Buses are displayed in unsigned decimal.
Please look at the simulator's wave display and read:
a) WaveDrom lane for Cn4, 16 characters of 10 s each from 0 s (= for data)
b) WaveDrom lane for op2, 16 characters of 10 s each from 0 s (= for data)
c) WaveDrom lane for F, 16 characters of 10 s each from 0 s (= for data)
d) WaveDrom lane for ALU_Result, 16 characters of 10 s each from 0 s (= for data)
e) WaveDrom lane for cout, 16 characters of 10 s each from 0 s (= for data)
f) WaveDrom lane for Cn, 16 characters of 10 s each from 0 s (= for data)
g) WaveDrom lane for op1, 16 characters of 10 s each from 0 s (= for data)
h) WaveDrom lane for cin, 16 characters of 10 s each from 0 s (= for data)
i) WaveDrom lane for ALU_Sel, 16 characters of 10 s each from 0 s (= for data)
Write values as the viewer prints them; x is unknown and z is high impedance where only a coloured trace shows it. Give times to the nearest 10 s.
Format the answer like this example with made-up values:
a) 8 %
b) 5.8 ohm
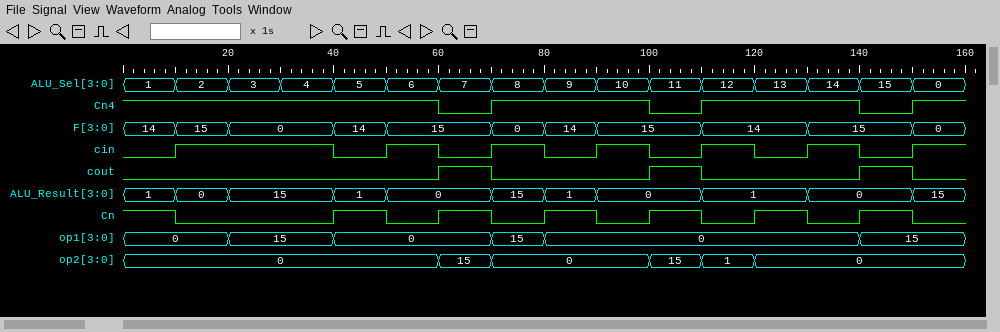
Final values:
a) {name: 'Cn4', wave: '1.....01..01..01'}
b) {name: 'op2', wave: '=.....==..===...', data: '0 15 0 15 1 0'}
c) {name: 'F', wave: '===.==.===.=.=.=', data: '14 15 0 14 15 0 14 15 14 15 0'}
d) {name: 'ALU_Result', wave: '===.==.===.=.=.=', data: '1 0 15 1 0 15 1 0 1 0 15'}
e) {name: 'cout', wave: '0.....10..10..10'}
f) {name: 'Cn', wave: '10..101010101010'}
g) {name: 'op1', wave: '=.=.=..==.....=.', data: '0 15 0 15 0 15'}
h) {name: 'cin', wave: '01..010101010101'}
i) {name: 'ALU_Sel', wave: '================', data: '1 2 3 4 5 6 7 8 9 10 11 12 13 14 15 0'}
